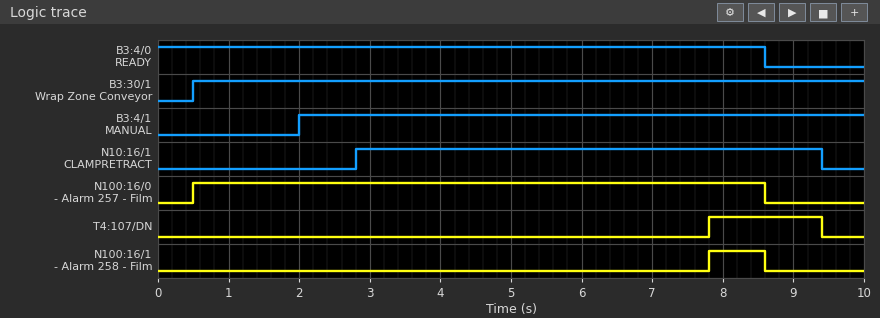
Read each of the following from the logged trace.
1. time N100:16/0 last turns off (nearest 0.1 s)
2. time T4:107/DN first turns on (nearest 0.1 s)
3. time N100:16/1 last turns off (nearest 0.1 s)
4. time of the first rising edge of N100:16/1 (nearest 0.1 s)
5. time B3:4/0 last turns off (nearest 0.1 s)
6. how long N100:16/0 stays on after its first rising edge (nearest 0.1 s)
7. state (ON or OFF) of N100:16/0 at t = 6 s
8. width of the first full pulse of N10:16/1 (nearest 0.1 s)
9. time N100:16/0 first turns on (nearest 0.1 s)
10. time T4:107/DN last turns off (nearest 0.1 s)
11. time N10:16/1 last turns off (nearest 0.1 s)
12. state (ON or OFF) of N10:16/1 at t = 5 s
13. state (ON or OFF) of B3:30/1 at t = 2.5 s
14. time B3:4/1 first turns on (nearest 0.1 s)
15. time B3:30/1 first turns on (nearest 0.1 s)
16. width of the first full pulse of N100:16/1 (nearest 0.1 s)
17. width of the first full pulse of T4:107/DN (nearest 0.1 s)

8.6 s
7.8 s
8.6 s
7.8 s
8.6 s
8.1 s
ON
6.6 s
0.5 s
9.4 s
9.4 s
ON
ON
2.0 s
0.5 s
0.8 s
1.6 s
